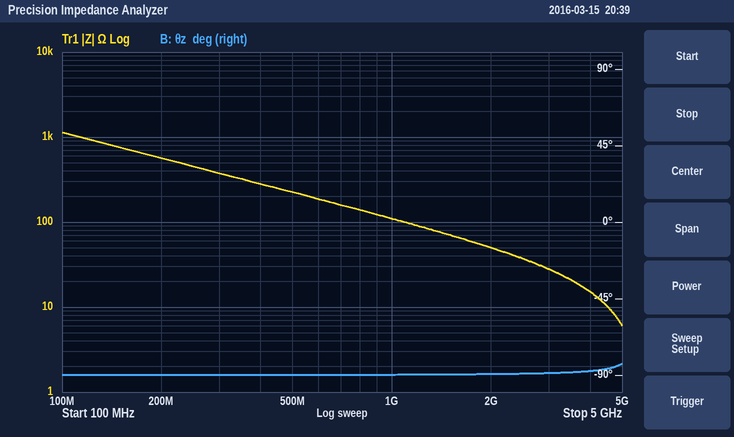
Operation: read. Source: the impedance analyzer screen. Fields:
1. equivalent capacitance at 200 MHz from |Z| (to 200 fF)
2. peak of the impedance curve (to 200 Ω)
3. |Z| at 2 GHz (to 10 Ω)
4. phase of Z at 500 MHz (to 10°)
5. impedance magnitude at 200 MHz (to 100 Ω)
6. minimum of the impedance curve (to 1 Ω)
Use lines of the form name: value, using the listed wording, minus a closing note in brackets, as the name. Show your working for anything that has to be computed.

equivalent capacitance at 200 MHz from |Z|: C = 1/(2π × 200 MHz × 600 Ω) ≈ 1.33 pF, so 1.4 pF to the nearest 200 fF
peak of the impedance curve: 1.2 kΩ
|Z| at 2 GHz: 50 Ω
phase of Z at 500 MHz: -90°
impedance magnitude at 200 MHz: 600 Ω
minimum of the impedance curve: 6 Ω
